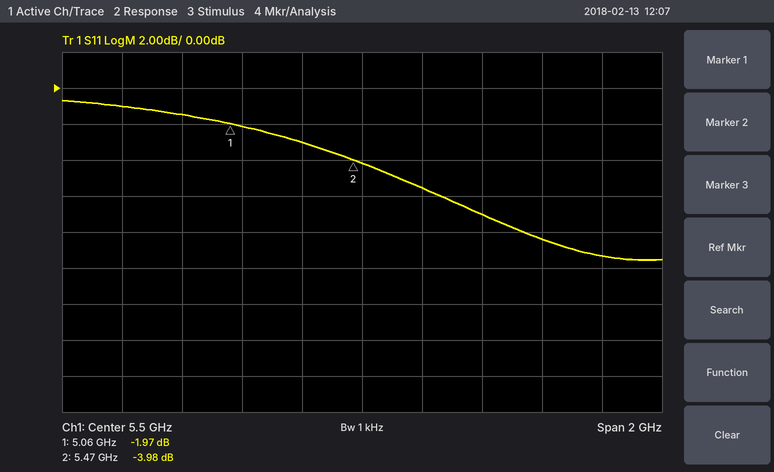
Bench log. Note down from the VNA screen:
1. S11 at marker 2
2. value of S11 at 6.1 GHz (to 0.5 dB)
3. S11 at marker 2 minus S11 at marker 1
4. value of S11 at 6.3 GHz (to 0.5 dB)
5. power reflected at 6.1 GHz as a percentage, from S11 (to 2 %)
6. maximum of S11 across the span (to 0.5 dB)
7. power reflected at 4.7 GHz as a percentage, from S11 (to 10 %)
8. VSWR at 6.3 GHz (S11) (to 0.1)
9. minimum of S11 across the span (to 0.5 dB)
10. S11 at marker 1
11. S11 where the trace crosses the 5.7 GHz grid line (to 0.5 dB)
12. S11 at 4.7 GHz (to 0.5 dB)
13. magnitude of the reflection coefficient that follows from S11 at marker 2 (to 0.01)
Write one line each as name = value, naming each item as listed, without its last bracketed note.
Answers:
S11 at marker 2 = -3.98 dB
value of S11 at 6.1 GHz = -8.5 dB
S11 at marker 2 minus S11 at marker 1 = -2.01 dB
value of S11 at 6.3 GHz = -9.5 dB
power reflected at 6.1 GHz as a percentage, from S11 = 14 %
maximum of S11 across the span = -0.5 dB
power reflected at 4.7 GHz as a percentage, from S11 = 80 %
VSWR at 6.3 GHz (S11) = 2.0
minimum of S11 across the span = -9.5 dB
S11 at marker 1 = -1.97 dB
S11 where the trace crosses the 5.7 GHz grid line = -5.5 dB
S11 at 4.7 GHz = -1.0 dB
magnitude of the reflection coefficient that follows from S11 at marker 2 = 0.63
